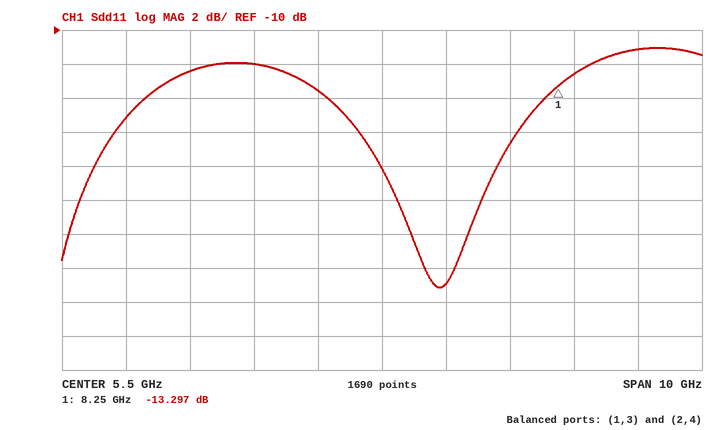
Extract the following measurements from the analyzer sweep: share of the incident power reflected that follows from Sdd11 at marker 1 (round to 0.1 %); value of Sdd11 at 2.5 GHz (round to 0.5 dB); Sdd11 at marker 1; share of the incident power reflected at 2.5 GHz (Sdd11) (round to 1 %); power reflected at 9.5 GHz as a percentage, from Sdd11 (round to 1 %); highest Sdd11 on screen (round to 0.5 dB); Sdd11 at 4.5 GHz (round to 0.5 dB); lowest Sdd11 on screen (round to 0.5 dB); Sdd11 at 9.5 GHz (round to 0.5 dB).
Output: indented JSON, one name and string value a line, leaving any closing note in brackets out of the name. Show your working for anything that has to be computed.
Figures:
{
  "share of the incident power reflected that follows from Sdd11 at marker 1": "10^(-13.297/10) ≈ 4.7 %",
  "value of Sdd11 at 2.5 GHz": "-12.5 dB",
  "Sdd11 at marker 1": "-13.297 dB",
  "share of the incident power reflected at 2.5 GHz (Sdd11)": "10^(-12.5/10) ≈ 6 %",
  "power reflected at 9.5 GHz as a percentage, from Sdd11": "10^(-11/10) ≈ 8 %",
  "highest Sdd11 on screen": "-11.0 dB",
  "Sdd11 at 4.5 GHz": "-13.5 dB",
  "lowest Sdd11 on screen": "-25.0 dB",
  "Sdd11 at 9.5 GHz": "-11.0 dB"
}
